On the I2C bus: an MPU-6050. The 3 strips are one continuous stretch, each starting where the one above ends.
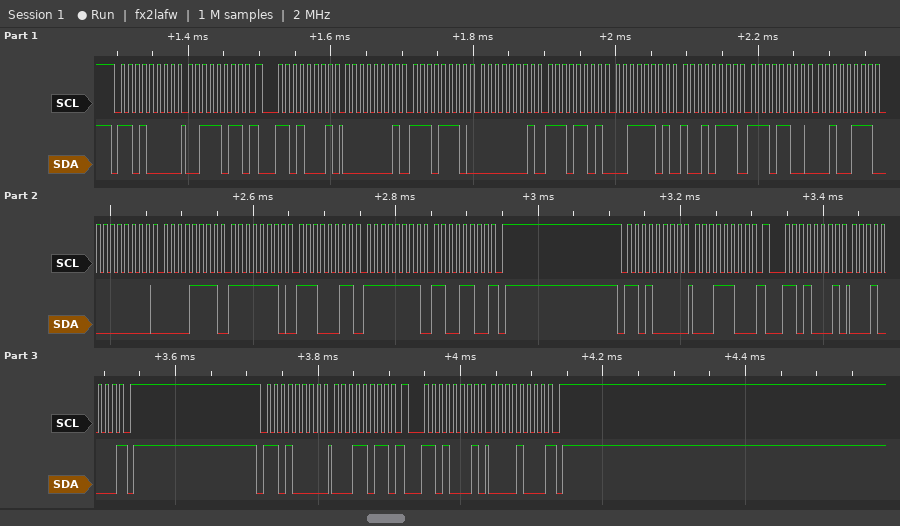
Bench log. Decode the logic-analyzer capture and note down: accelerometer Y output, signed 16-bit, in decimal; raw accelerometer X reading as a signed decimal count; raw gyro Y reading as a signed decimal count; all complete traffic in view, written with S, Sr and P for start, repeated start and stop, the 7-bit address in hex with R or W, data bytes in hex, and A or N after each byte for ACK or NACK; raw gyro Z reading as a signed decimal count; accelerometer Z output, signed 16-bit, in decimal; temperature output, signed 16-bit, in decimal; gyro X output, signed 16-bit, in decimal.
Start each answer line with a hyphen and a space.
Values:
- 493
- 494
- -285
- S 68W A 3B A Sr 68R A 01 A EE A 01 A ED A 3D A 97 A EC A 27 A 00 A 0F A FE A E3 A FF A CC N P S 68W A 1C A Sr 68R A 10 N P S 68W A 1B A Sr 68R A 08 N P
- -52
- 15767
- -5081
- 15
